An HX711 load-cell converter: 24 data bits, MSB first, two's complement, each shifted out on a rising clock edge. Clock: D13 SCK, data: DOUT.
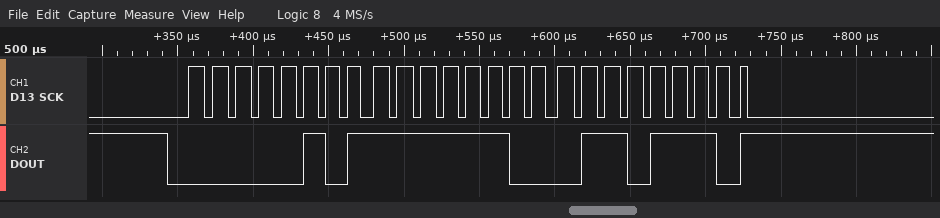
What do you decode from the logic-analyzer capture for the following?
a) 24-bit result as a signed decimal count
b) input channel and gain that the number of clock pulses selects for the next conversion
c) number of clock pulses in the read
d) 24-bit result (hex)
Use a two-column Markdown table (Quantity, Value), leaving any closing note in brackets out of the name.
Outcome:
| Quantity | Value |
|---|---|
| 24-bit result as a signed decimal count | 392302 |
| input channel and gain that the number of clock pulses selects for the next conversion | channel A, gain 128 |
| number of clock pulses in the read | 25 |
| 24-bit result | 0x05FC6E |
